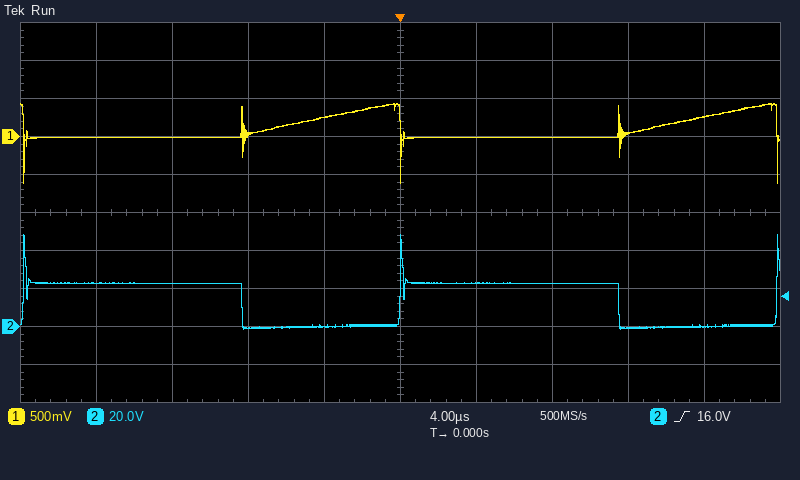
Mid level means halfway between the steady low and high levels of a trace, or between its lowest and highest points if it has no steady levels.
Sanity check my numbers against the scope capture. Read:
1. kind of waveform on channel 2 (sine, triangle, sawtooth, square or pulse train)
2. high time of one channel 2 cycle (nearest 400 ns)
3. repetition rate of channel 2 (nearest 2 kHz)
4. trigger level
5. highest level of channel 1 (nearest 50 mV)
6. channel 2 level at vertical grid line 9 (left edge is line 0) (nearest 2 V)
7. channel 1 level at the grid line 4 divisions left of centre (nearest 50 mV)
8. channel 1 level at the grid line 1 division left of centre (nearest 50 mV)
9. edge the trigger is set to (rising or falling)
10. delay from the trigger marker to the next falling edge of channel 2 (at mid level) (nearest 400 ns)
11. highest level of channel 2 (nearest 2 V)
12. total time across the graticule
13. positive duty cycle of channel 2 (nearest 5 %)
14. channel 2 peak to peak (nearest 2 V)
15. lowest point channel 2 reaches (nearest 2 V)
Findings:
pulse train
11.6 µs
50 kHz
16.0 V
450 mV
0 V
0 mV
250 mV
rising
11.6 µs
48 V
40 µs
60 %
50 V
-2 V
